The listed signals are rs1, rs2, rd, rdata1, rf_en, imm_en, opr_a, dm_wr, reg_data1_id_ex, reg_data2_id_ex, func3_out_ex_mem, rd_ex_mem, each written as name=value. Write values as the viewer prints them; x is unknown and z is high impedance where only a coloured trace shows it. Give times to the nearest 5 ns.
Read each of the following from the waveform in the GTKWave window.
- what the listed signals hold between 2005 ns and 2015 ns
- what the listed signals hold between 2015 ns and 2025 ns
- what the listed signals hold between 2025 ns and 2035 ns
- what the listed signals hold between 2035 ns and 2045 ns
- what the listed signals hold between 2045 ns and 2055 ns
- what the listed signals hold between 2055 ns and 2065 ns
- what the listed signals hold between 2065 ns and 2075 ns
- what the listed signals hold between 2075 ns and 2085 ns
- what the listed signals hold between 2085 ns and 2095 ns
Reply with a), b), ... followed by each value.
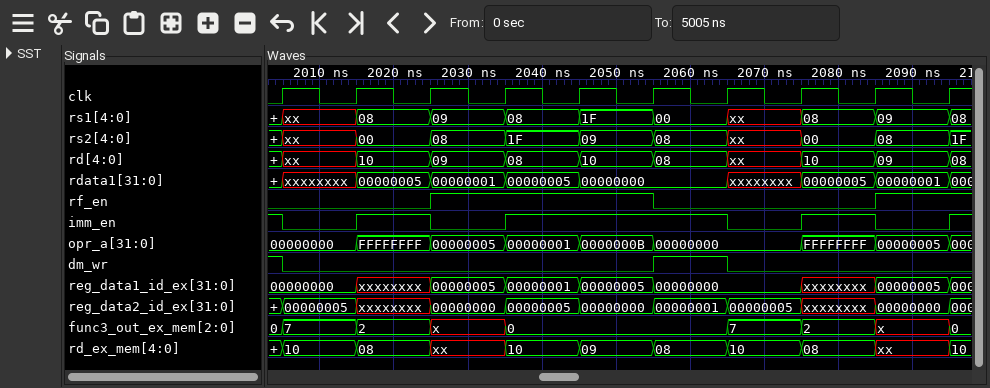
a) rs1=xx, rs2=xx, rd=xx, rdata1=xxxxxxxx, rf_en=0, imm_en=0, opr_a=00000000, dm_wr=0, reg_data1_id_ex=00000000, reg_data2_id_ex=00000005, func3_out_ex_mem=7, rd_ex_mem=10
b) rs1=08, rs2=00, rd=10, rdata1=00000005, rf_en=0, imm_en=1, opr_a=FFFFFFFF, dm_wr=0, reg_data1_id_ex=xxxxxxxx, reg_data2_id_ex=xxxxxxxx, func3_out_ex_mem=2, rd_ex_mem=08
c) rs1=09, rs2=08, rd=09, rdata1=00000001, rf_en=1, imm_en=0, opr_a=00000005, dm_wr=0, reg_data1_id_ex=00000005, reg_data2_id_ex=00000000, func3_out_ex_mem=x, rd_ex_mem=xx
d) rs1=08, rs2=1F, rd=08, rdata1=00000005, rf_en=1, imm_en=1, opr_a=00000001, dm_wr=0, reg_data1_id_ex=00000001, reg_data2_id_ex=00000005, func3_out_ex_mem=0, rd_ex_mem=10
e) rs1=1F, rs2=09, rd=10, rdata1=00000000, rf_en=1, imm_en=1, opr_a=0000000B, dm_wr=0, reg_data1_id_ex=00000005, reg_data2_id_ex=00000000, func3_out_ex_mem=0, rd_ex_mem=09
f) rs1=00, rs2=08, rd=08, rdata1=00000000, rf_en=0, imm_en=1, opr_a=00000000, dm_wr=1, reg_data1_id_ex=00000000, reg_data2_id_ex=00000001, func3_out_ex_mem=0, rd_ex_mem=08
g) rs1=xx, rs2=xx, rd=xx, rdata1=xxxxxxxx, rf_en=0, imm_en=0, opr_a=00000000, dm_wr=0, reg_data1_id_ex=00000000, reg_data2_id_ex=00000005, func3_out_ex_mem=7, rd_ex_mem=10
h) rs1=08, rs2=00, rd=10, rdata1=00000005, rf_en=0, imm_en=1, opr_a=FFFFFFFF, dm_wr=0, reg_data1_id_ex=xxxxxxxx, reg_data2_id_ex=xxxxxxxx, func3_out_ex_mem=2, rd_ex_mem=08
i) rs1=09, rs2=08, rd=09, rdata1=00000001, rf_en=1, imm_en=0, opr_a=00000005, dm_wr=0, reg_data1_id_ex=00000005, reg_data2_id_ex=00000000, func3_out_ex_mem=x, rd_ex_mem=xx
